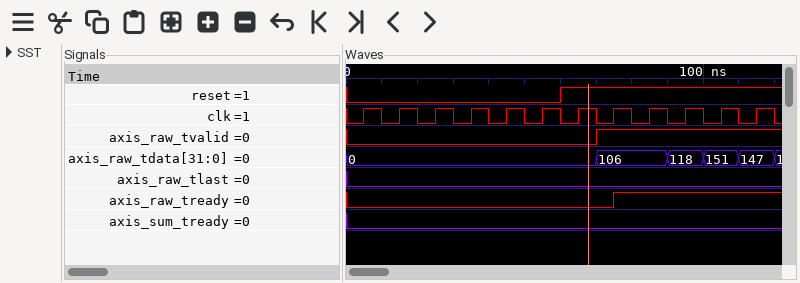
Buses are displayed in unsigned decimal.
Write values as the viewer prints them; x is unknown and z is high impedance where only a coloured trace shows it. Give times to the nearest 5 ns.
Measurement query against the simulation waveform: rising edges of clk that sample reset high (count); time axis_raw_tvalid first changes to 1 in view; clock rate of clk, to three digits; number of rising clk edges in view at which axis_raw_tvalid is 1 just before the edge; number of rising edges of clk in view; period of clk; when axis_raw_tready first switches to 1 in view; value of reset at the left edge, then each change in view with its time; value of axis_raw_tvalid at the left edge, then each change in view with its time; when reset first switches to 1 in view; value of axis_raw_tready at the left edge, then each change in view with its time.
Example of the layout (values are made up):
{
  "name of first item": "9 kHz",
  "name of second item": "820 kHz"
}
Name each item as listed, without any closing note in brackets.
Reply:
{
  "rising edges of clk that sample reset high": "6",
  "time axis_raw_tvalid first changes to 1 in view": "70 ns",
  "clock rate of clk, to three digits": "100 MHz",
  "number of rising clk edges in view at which axis_raw_tvalid is 1 just before the edge": "5",
  "number of rising edges of clk in view": "12",
  "period of clk": "10 ns",
  "when axis_raw_tready first switches to 1 in view": "75 ns",
  "value of reset at the left edge, then each change in view with its time": "0, 1 at 60 ns",
  "value of axis_raw_tvalid at the left edge, then each change in view with its time": "0, 1 at 70 ns",
  "when reset first switches to 1 in view": "60 ns",
  "value of axis_raw_tready at the left edge, then each change in view with its time": "0, 1 at 75 ns"
}
